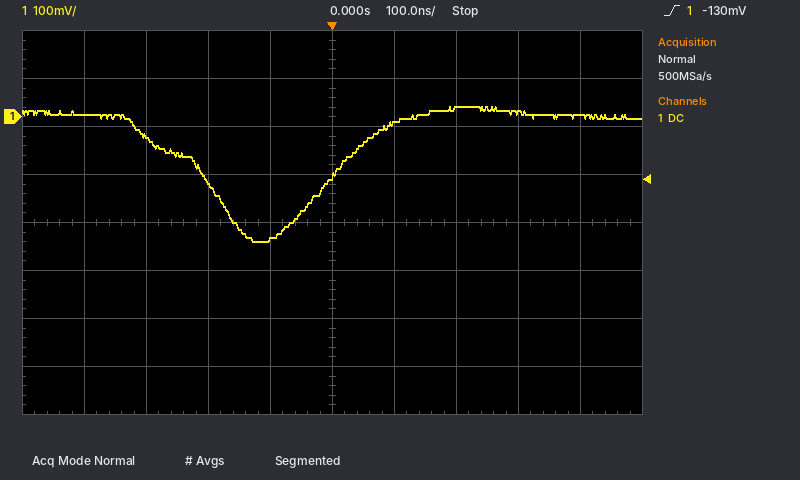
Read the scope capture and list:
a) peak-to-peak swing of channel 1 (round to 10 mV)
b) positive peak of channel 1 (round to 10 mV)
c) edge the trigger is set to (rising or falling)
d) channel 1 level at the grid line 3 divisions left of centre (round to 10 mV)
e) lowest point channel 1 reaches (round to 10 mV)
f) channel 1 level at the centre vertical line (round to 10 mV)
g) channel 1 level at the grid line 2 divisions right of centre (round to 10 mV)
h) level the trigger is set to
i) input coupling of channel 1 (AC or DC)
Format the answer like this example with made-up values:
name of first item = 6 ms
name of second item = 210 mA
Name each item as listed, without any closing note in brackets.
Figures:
peak-to-peak swing of channel 1 = 280 mV
positive peak of channel 1 = 20 mV
edge the trigger is set to = rising
channel 1 level at the grid line 3 divisions left of centre = -40 mV
lowest point channel 1 reaches = -260 mV
channel 1 level at the centre vertical line = -120 mV
channel 1 level at the grid line 2 divisions right of centre = 20 mV
level the trigger is set to = -130 mV
input coupling of channel 1 = DC
